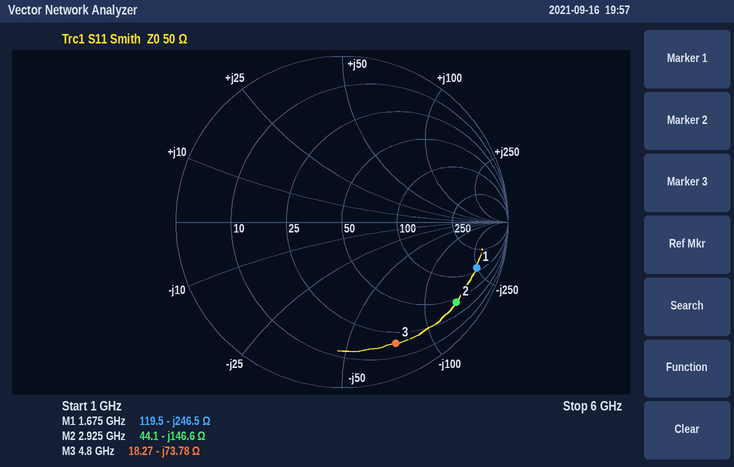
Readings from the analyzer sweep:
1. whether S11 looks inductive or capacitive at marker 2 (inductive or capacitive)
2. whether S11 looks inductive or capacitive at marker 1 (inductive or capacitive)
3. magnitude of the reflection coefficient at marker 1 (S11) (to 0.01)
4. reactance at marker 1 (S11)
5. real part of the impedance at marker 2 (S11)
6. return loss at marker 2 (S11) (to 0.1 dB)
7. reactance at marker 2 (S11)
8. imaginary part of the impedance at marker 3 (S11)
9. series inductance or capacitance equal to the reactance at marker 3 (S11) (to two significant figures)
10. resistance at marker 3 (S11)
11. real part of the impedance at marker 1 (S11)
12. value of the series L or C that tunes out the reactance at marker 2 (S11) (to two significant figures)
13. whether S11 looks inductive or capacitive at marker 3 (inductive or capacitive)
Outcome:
capacitive
capacitive
0.86
-246.5 Ω
44.1 Ω
1.5 dB
-146.6 Ω
-73.78 Ω
450 fF
18.27 Ω
119.5 Ω
8.0 nH
capacitive
